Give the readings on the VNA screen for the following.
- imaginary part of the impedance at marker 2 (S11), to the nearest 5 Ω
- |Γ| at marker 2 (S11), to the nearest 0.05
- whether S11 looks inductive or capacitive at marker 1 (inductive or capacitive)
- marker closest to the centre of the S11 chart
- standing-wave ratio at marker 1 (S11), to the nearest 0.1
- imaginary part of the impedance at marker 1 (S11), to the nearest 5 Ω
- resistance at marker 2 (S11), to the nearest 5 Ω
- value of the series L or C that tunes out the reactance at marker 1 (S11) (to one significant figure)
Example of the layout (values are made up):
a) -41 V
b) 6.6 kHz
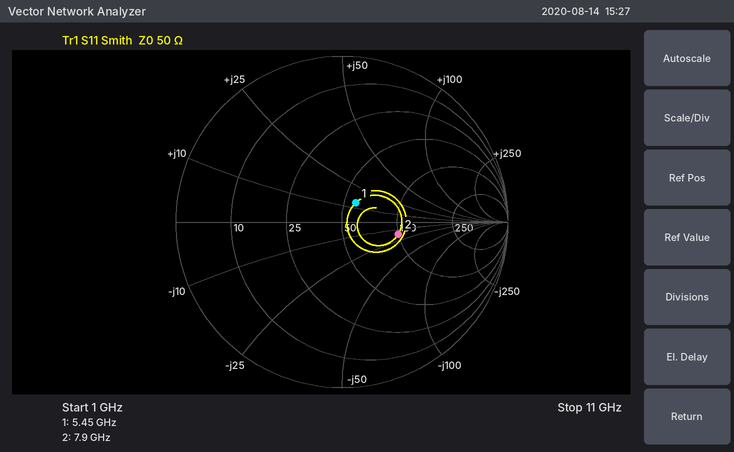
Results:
a) -15 Ω
b) 0.35
c) inductive
d) marker 1
e) 1.3
f) +15 Ω
g) 100 Ω
h) 2 pF
